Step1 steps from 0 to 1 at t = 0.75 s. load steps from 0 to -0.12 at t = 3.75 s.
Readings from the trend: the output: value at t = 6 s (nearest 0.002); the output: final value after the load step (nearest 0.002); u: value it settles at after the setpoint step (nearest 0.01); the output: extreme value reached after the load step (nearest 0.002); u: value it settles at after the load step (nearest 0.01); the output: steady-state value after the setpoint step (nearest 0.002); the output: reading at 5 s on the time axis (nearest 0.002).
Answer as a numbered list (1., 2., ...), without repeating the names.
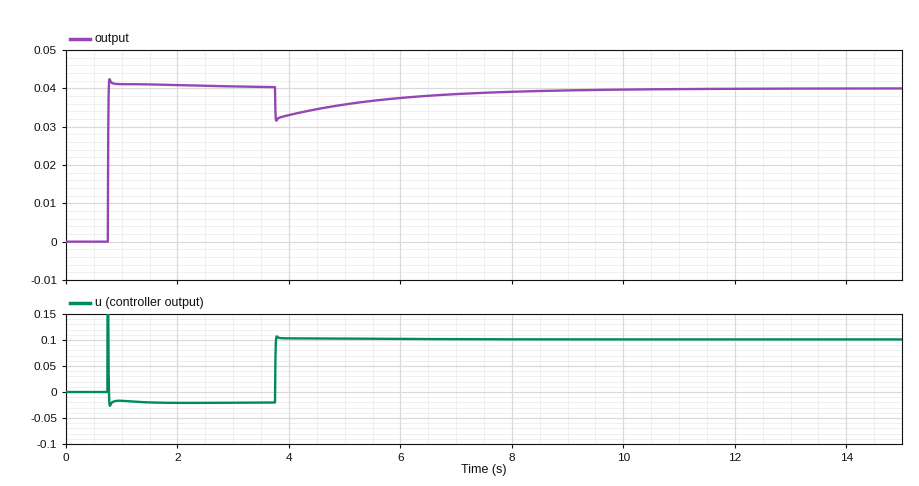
1. 0.038
2. 0.040
3. -0.02
4. 0.032
5. 0.10
6. 0.040
7. 0.036
